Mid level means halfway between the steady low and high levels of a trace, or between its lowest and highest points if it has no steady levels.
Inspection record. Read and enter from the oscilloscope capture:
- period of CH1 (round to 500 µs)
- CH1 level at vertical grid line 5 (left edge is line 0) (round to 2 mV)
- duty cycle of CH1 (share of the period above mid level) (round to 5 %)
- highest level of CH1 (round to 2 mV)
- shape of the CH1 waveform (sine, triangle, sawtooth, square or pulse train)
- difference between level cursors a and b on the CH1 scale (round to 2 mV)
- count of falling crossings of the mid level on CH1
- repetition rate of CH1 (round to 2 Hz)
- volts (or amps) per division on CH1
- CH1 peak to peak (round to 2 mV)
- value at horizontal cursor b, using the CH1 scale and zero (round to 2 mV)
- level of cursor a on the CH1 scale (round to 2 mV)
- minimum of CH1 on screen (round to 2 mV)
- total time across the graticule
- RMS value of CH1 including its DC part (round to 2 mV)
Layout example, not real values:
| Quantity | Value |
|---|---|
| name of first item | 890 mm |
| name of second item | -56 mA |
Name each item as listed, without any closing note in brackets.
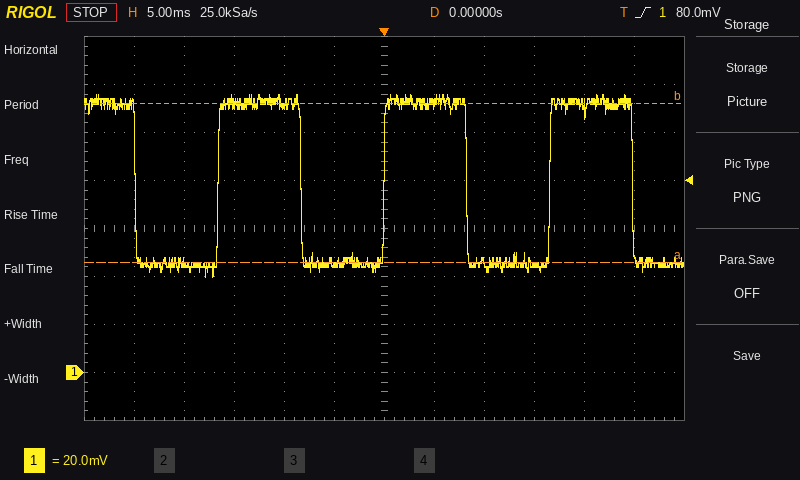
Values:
| Quantity | Value |
|---|---|
| period of CH1 | 16.5 ms |
| CH1 level at vertical grid line 5 (left edge is line 0) | 46 mV |
| duty cycle of CH1 (share of the period above mid level) | 50 % |
| highest level of CH1 | 116 mV |
| shape of the CH1 waveform | square |
| difference between level cursors a and b on the CH1 scale | 66 mV |
| count of falling crossings of the mid level on CH1 | 4 |
| repetition rate of CH1 | 60 Hz |
| volts (or amps) per division on CH1 | 20 mV |
| CH1 peak to peak | 76 mV |
| value at horizontal cursor b, using the CH1 scale and zero | 112 mV |
| level of cursor a on the CH1 scale | 46 mV |
| minimum of CH1 on screen | 40 mV |
| total time across the graticule | 60 ms |
| RMS value of CH1 including its DC part | 86 mV |
